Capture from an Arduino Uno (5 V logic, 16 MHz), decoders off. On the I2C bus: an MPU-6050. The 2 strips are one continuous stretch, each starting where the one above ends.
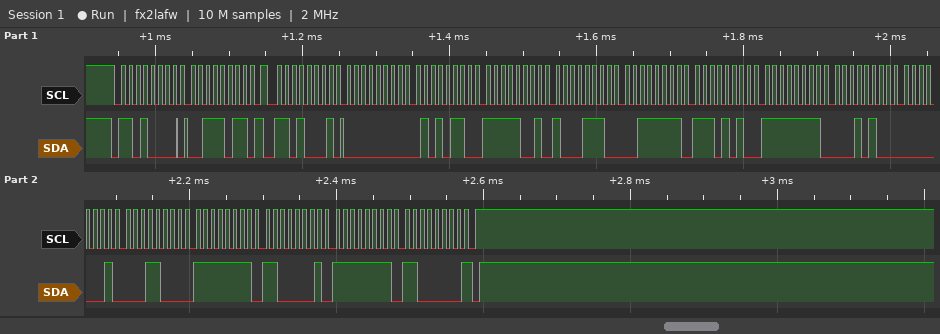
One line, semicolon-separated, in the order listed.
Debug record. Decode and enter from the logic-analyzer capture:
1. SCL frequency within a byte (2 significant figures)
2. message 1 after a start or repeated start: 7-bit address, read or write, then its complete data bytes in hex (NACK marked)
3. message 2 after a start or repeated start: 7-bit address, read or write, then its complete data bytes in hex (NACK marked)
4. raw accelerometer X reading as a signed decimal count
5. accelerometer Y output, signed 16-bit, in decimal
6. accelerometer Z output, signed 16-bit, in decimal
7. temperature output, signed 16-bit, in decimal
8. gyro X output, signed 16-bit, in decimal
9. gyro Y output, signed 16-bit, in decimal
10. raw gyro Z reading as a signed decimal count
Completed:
100 kHz; 0x68 write: 3B; 0x68 read: 00 56 F9 8E 3F EA FF 14 01 18 FF C1 FF C0 NACK; 86; -1650; 16362; -236; 280; -63; -64
